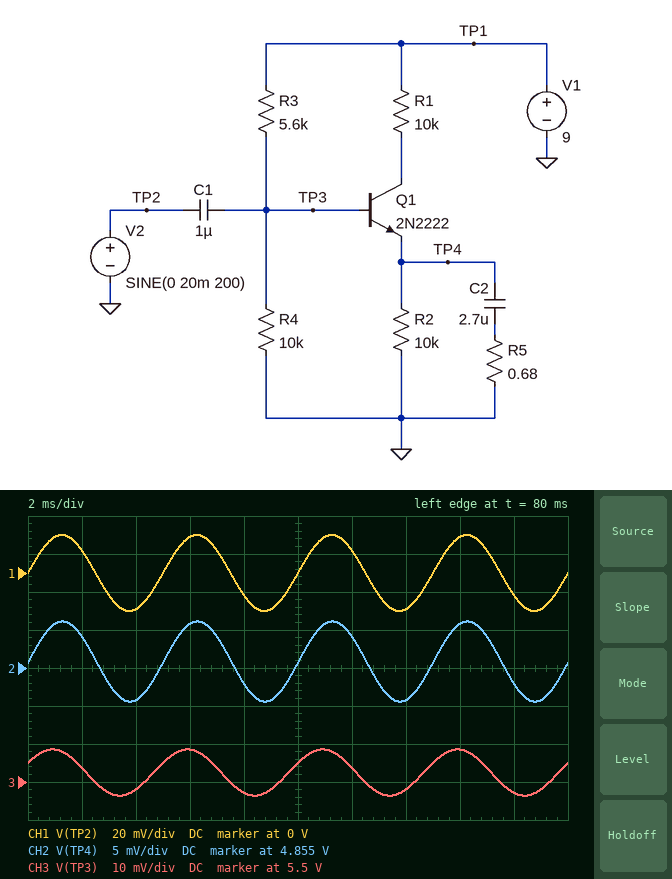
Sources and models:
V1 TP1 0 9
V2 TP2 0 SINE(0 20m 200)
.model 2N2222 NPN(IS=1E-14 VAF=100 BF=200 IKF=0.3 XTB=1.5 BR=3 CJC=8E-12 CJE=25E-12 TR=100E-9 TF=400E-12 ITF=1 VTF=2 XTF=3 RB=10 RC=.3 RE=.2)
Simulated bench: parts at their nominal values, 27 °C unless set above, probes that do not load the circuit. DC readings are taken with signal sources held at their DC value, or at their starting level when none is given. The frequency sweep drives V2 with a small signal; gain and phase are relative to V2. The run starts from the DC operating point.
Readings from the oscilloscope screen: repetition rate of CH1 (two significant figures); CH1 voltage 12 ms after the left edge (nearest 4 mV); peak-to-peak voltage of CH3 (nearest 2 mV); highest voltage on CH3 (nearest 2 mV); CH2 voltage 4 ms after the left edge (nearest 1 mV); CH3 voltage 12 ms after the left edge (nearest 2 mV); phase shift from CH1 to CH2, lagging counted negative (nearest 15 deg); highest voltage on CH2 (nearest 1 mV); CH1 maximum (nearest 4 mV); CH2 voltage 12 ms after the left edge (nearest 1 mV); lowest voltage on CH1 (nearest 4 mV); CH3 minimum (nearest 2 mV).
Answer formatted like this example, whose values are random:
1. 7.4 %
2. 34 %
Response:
1. 200 Hz
2. 12 mV
3. 12 mV
4. 5.508 V
5. 4.851 V
6. 5.504 V
7. 0 deg
8. 4.861 V
9. 20 mV
10. 4.859 V
11. -20 mV
12. 5.496 V
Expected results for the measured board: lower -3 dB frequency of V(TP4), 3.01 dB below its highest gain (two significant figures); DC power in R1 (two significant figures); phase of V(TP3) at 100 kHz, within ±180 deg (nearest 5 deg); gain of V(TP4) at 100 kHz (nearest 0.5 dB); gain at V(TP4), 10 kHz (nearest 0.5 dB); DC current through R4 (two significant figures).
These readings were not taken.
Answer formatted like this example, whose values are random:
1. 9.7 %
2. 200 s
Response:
1. 20 Hz
2. 1.7 mW
3. 0 deg
4. -44.5 dB
5. -28.5 dB
6. 550 µA
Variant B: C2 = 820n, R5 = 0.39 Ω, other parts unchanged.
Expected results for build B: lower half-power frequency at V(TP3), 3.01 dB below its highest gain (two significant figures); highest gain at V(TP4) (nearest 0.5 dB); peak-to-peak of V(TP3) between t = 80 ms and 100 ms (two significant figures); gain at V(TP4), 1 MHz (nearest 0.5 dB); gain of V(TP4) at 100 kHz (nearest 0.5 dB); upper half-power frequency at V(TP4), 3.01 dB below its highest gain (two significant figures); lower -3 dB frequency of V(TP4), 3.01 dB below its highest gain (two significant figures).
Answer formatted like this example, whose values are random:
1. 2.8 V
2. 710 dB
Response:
1. 1.4 kHz
2. -5.5 dB
3. 22 mV
4. -45.5 dB
5. -37.5 dB
6. 2.4 kHz
7. 40 Hz
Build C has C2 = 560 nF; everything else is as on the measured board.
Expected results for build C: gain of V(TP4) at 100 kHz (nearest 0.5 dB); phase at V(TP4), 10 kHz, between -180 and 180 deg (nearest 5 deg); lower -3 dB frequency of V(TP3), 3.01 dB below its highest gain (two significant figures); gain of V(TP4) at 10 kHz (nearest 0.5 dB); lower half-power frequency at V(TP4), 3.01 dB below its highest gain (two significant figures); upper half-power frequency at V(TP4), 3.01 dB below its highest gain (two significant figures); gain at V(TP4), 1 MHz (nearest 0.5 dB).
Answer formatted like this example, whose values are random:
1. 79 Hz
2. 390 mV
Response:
1. -34.5 dB
2. -70 deg
3. 1.1 kHz
4. -15.0 dB
5. 47 Hz
6. 3.0 kHz
7. -41.0 dB
